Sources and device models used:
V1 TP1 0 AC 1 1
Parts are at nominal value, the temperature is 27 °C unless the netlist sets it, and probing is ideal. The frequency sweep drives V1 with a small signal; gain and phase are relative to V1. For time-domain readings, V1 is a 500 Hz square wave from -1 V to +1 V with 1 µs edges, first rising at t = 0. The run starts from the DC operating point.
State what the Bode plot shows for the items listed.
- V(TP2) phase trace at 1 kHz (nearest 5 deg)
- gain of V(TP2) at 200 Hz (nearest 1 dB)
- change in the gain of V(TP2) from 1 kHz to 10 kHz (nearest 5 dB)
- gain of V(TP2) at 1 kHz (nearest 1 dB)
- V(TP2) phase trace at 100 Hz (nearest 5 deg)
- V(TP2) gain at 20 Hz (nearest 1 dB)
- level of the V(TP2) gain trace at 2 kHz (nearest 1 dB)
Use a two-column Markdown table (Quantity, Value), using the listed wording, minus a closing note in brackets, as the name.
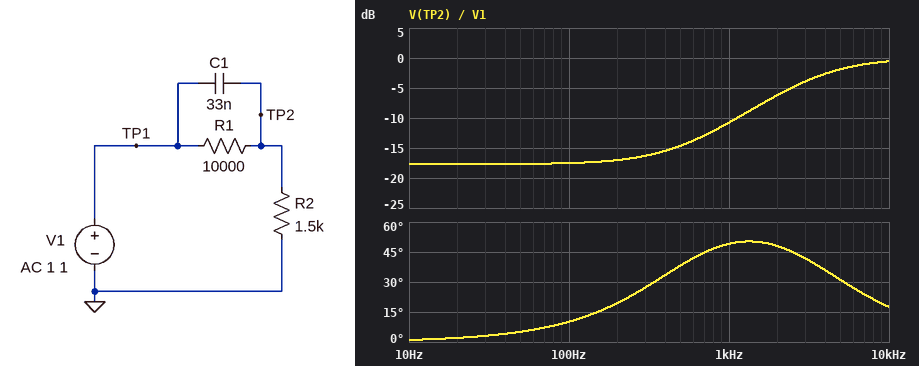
| Quantity | Value |
|---|---|
| V(TP2) phase trace at 1 kHz | 50 deg |
| gain of V(TP2) at 200 Hz | -17 dB |
| change in the gain of V(TP2) from 1 kHz to 10 kHz | 10 dB |
| gain of V(TP2) at 1 kHz | -11 dB |
| V(TP2) phase trace at 100 Hz | 10 deg |
| V(TP2) gain at 20 Hz | -18 dB |
| level of the V(TP2) gain trace at 2 kHz | -6 dB |
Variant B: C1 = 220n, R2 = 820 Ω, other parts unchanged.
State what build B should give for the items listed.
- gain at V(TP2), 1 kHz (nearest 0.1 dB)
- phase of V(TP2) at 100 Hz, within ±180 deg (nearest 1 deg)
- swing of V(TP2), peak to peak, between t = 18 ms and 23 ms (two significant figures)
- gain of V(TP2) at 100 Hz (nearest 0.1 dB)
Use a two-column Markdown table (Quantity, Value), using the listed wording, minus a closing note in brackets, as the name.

| Quantity | Value |
|---|---|
| gain at V(TP2), 1 kHz | -2.8 dB |
| phase of V(TP2) at 100 Hz, within ±180 deg | 48 deg |
| swing of V(TP2), peak to peak, between t = 18 ms and 23 ms | 3.8 V |
| gain of V(TP2) at 100 Hz | -17.8 dB |
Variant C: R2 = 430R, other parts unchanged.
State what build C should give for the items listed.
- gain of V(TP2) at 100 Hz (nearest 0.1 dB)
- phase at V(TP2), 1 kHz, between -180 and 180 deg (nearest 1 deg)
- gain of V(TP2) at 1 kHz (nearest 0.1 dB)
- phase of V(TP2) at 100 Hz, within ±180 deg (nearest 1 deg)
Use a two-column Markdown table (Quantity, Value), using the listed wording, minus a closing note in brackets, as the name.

| Quantity | Value |
|---|---|
| gain of V(TP2) at 100 Hz | -27.5 dB |
| phase at V(TP2), 1 kHz, between -180 and 180 deg | 59 deg |
| gain of V(TP2) at 1 kHz | -20.5 dB |
| phase of V(TP2) at 100 Hz, within ±180 deg | 11 deg |
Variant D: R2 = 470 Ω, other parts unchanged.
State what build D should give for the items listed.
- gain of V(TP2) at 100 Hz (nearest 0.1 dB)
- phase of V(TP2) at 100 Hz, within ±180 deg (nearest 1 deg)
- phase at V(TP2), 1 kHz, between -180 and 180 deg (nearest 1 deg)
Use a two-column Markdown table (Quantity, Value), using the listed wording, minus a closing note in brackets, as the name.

| Quantity | Value |
|---|---|
| gain of V(TP2) at 100 Hz | -26.8 dB |
| phase of V(TP2) at 100 Hz, within ±180 deg | 11 deg |
| phase at V(TP2), 1 kHz, between -180 and 180 deg | 59 deg |
